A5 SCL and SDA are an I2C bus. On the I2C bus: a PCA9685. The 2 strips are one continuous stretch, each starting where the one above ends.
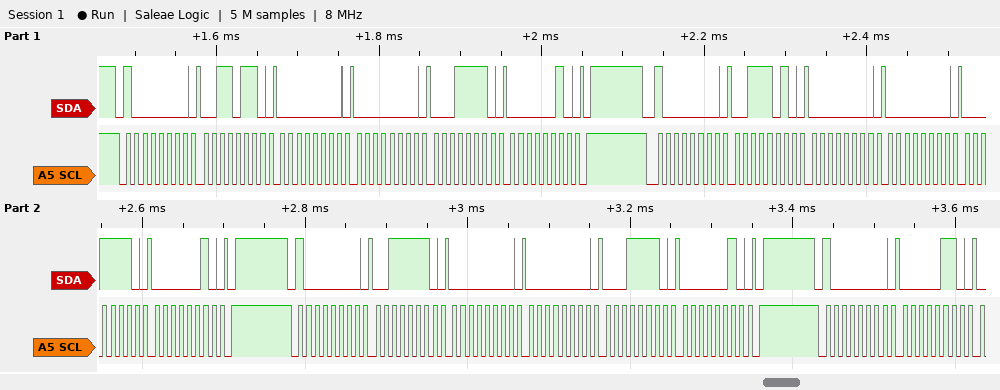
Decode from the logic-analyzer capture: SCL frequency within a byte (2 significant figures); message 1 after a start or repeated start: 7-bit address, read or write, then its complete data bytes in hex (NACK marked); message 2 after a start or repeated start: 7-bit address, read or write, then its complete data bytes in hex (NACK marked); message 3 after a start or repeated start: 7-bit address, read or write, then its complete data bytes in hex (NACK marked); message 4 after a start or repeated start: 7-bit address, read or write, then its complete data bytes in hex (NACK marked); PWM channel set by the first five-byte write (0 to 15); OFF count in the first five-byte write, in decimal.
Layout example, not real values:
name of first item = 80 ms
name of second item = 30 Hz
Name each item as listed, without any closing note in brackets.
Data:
SCL frequency within a byte = 100 kHz
message 1 after a start or repeated start: 7-bit address, read or write, then its complete data bytes in hex = 0x40 write: 36 00 00 1E 02
message 2 after a start or repeated start: 7-bit address, read or write, then its complete data bytes in hex = 0x40 write: 3A 00 00 1E 02
message 3 after a start or repeated start: 7-bit address, read or write, then its complete data bytes in hex = 0x40 write: 3E 00 00 1E 02
message 4 after a start or repeated start: 7-bit address, read or write, then its complete data bytes in hex = 0x40 write: 06
PWM channel set by the first five-byte write = 12
OFF count in the first five-byte write, in decimal = 542
